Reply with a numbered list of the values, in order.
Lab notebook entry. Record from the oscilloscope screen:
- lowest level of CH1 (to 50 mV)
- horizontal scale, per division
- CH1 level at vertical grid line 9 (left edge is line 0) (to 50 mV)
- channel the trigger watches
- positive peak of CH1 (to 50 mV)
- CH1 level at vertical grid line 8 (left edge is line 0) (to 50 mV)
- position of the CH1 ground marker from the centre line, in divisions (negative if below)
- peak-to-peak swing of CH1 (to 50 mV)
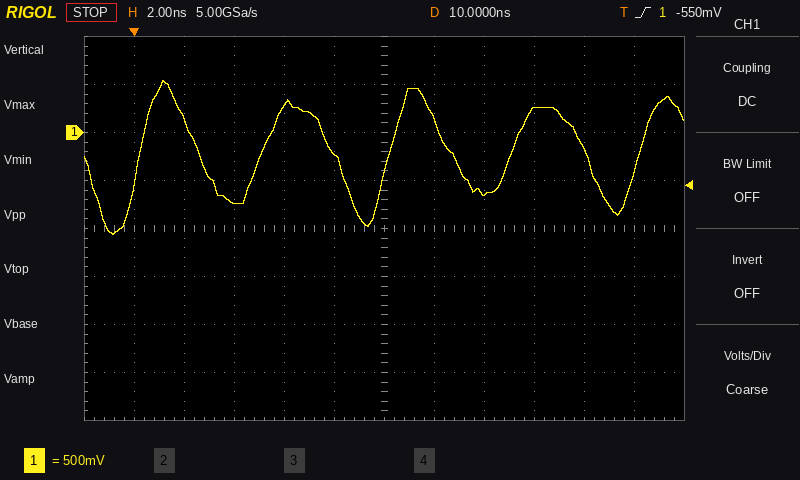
1. -1.05 V
2. 2 ns
3. 250 mV
4. CH1
5. 550 mV
6. -650 mV
7. +2.0 div
8. 1.60 V
